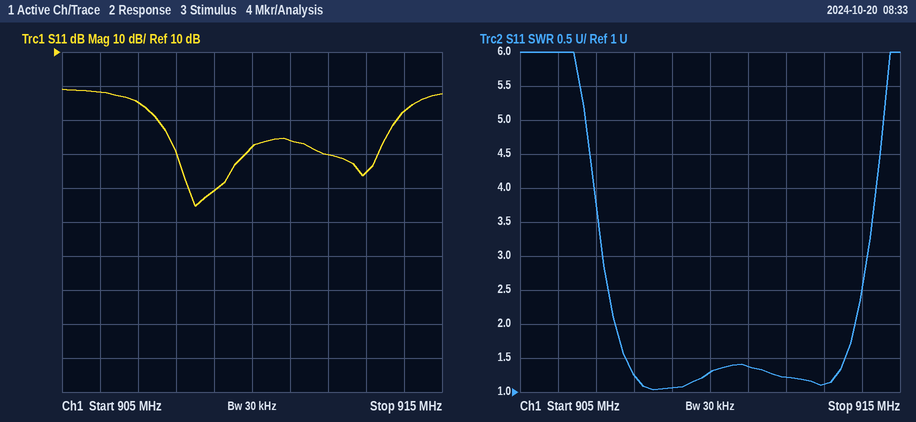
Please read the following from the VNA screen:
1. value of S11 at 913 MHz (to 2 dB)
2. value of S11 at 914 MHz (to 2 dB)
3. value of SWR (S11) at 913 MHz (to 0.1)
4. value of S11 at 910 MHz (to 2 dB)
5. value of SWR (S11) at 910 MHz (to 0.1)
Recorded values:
-26 dB
-8 dB
1.1
-18 dB
1.3
